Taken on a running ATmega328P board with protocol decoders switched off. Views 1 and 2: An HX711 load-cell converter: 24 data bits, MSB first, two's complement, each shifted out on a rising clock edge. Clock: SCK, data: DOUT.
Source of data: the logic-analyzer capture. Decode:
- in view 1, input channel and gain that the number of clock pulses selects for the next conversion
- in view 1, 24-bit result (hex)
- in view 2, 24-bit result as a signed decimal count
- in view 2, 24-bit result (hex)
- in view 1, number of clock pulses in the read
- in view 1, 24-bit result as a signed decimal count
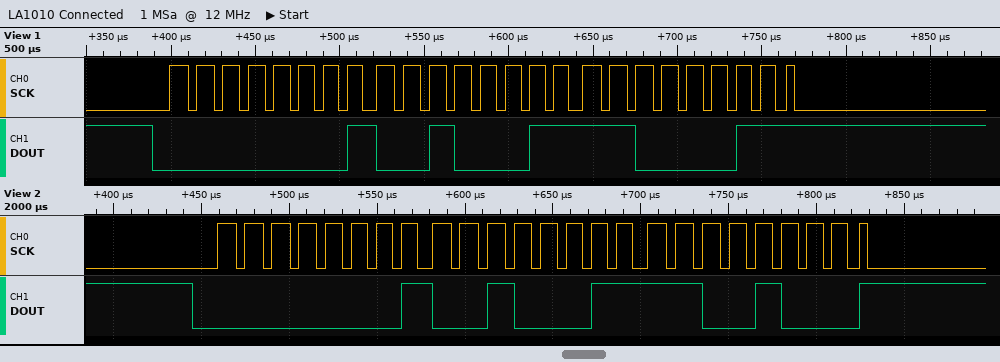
channel A, gain 128
0x0123C3
74696
0x0123C8
25
74691
